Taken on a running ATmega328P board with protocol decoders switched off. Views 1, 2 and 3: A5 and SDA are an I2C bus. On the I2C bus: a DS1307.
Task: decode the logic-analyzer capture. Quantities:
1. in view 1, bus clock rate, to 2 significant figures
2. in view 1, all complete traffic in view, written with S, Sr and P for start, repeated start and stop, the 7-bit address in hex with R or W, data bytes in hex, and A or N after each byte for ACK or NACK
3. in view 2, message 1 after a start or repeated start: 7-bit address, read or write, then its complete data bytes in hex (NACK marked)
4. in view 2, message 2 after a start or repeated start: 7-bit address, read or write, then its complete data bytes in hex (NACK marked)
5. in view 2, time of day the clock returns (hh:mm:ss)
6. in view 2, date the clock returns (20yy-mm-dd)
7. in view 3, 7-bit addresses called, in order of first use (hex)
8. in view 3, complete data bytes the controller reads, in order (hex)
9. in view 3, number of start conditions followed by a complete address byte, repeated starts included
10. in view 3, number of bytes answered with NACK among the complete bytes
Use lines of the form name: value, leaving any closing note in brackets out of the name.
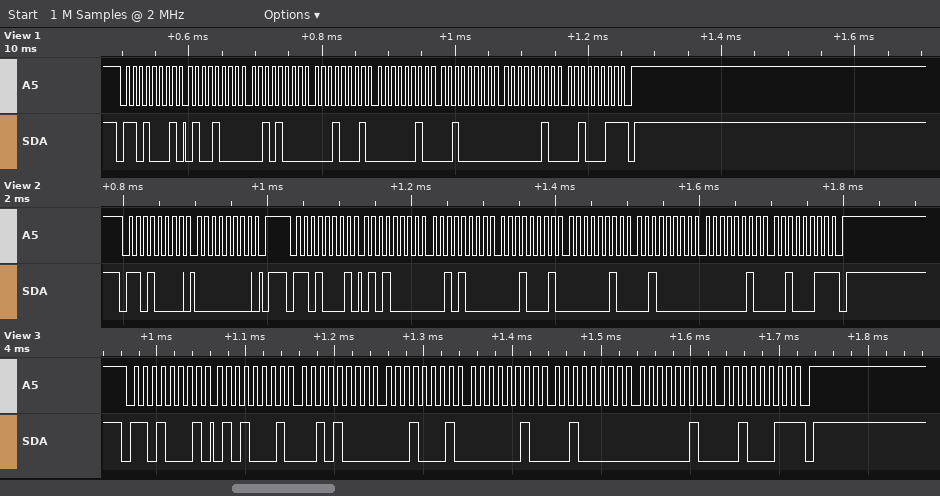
in view 1, bus clock rate, to 2 significant figures: 100 kHz
in view 1, all complete traffic in view, written with S, Sr and P for start, repeated start and stop, the 7-bit address in hex with R or W, data bytes in hex, and A or N after each byte for ACK or NACK: S 68R A 48 A 28 A 11 A 02 A 20 A 02 A 23 N P
in view 2, message 1 after a start or repeated start: 7-bit address, read or write, then its complete data bytes in hex: 0x68 write: 00
in view 2, message 2 after a start or repeated start: 7-bit address, read or write, then its complete data bytes in hex: 0x68 read: 50 28 11 02 20 02 23 NACK
in view 2, time of day the clock returns: 11:28:50
in view 2, date the clock returns: 2023-02-20
in view 3, 7-bit addresses called, in order of first use: 0x68
in view 3, complete data bytes the controller reads, in order: 51 28 11 02 20 02 23
in view 3, number of start conditions followed by a complete address byte, repeated starts included: 1
in view 3, number of bytes answered with NACK among the complete bytes: 1
